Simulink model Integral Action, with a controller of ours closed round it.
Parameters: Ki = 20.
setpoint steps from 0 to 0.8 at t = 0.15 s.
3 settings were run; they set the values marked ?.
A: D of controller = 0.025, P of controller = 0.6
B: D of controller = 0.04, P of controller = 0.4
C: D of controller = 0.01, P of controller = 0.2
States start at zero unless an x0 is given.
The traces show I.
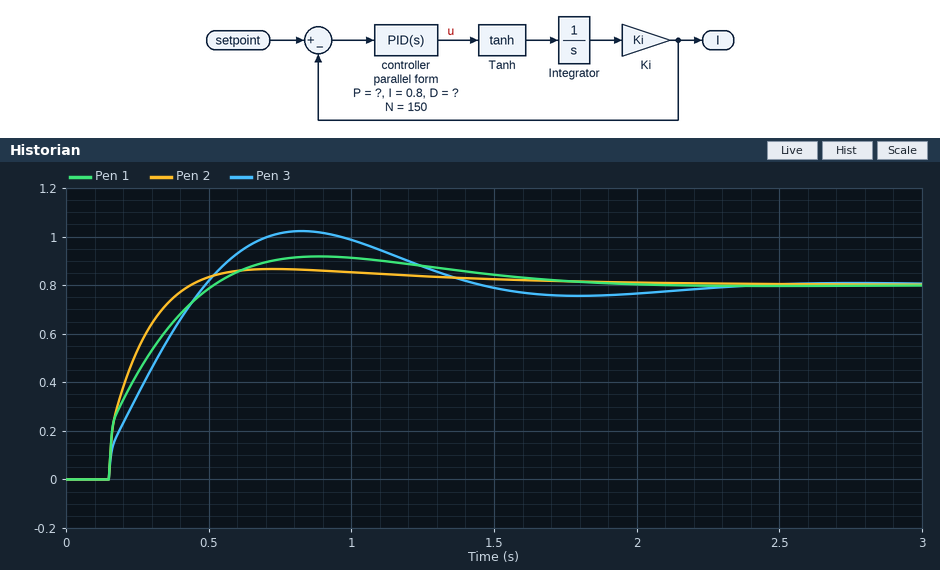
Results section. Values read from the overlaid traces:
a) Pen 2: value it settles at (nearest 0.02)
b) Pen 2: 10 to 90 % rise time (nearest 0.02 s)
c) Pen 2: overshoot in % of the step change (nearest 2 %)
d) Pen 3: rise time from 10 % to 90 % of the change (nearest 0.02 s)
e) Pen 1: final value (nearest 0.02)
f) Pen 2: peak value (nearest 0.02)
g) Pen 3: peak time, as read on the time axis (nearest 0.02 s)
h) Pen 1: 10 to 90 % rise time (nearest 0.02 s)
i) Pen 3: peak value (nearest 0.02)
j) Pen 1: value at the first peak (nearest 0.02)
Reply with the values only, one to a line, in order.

0.80
0.20 s
8 %
0.28 s
0.80
0.86
0.82 s
0.28 s
1.02
0.92
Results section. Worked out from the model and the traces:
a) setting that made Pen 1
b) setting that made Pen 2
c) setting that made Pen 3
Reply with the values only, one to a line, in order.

B
A
C
